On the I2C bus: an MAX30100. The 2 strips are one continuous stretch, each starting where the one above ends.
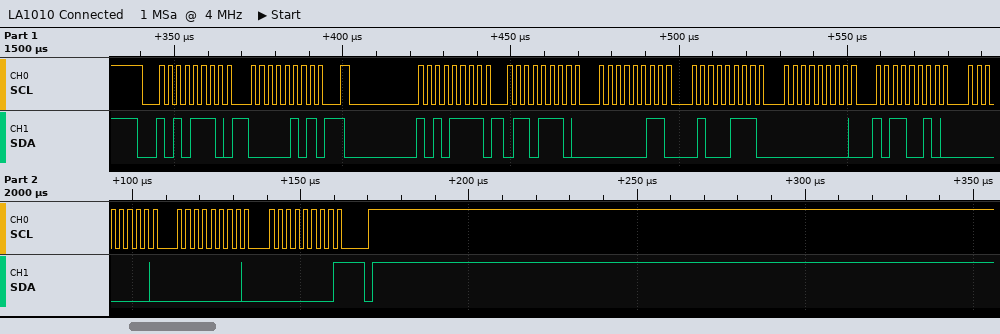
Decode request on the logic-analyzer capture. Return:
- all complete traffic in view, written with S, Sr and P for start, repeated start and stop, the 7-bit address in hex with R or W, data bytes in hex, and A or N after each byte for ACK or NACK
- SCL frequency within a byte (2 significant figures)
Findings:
S 57W A 05 A Sr 57R A 6E A 03 A 47 A 00 A B2 A 00 A 00 A 00 N P
400 kHz
